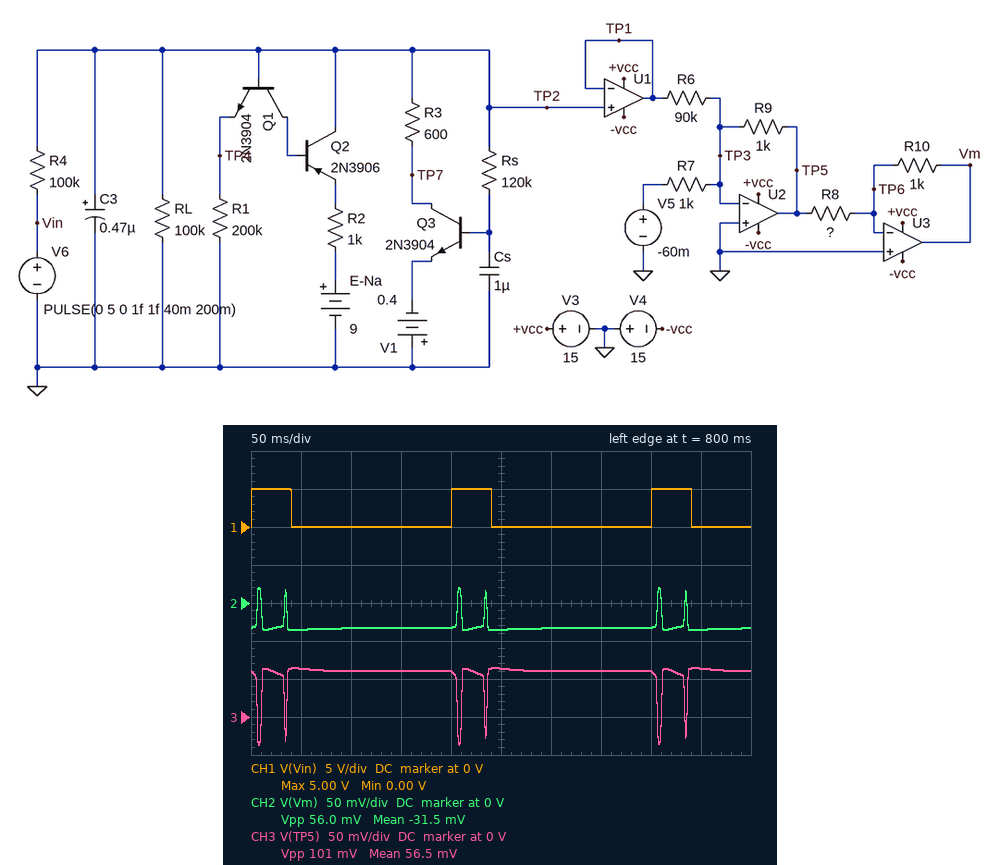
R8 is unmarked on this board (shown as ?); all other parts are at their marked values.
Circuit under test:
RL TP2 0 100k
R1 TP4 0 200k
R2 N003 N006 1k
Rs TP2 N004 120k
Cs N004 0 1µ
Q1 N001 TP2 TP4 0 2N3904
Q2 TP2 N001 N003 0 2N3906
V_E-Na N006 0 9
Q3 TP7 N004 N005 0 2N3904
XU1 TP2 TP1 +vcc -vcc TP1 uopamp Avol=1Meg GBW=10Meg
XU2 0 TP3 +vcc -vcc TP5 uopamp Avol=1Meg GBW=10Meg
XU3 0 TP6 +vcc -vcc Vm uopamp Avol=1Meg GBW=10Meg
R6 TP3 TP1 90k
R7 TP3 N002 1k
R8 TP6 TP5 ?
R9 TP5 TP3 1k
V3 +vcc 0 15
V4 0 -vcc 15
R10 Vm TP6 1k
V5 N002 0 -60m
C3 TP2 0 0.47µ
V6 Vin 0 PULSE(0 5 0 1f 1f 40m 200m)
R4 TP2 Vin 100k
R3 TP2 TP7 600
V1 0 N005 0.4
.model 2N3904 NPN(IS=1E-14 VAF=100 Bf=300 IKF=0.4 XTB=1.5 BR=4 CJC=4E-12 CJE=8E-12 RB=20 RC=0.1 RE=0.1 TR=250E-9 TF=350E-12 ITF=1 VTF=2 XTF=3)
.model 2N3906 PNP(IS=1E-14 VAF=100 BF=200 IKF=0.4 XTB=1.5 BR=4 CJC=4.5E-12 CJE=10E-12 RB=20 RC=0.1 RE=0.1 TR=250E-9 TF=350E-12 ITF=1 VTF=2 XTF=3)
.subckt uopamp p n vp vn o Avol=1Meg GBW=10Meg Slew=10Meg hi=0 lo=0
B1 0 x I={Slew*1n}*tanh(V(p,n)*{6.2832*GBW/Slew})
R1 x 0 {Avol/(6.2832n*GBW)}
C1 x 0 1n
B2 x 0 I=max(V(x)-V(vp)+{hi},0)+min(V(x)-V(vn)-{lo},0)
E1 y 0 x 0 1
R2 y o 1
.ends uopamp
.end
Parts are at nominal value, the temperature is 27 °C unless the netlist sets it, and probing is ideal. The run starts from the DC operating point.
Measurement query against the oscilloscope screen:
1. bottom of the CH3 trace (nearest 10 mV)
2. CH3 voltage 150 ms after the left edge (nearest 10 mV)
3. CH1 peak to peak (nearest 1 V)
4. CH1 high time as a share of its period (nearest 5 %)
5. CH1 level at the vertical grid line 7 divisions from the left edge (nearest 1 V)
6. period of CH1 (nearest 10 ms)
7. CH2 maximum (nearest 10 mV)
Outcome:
-40 mV
60 mV
5 V
20 %
0 V
200 ms
20 mV
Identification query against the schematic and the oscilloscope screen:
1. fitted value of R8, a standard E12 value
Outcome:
1.8 kΩ
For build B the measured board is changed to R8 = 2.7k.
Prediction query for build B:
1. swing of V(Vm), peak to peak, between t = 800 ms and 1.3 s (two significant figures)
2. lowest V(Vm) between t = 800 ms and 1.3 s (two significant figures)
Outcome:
37 mV
-24 mV
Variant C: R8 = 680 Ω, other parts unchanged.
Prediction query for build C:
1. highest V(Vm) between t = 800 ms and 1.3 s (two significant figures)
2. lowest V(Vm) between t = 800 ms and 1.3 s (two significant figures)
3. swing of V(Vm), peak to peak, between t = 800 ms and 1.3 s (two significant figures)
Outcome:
53 mV
-94 mV
150 mV
